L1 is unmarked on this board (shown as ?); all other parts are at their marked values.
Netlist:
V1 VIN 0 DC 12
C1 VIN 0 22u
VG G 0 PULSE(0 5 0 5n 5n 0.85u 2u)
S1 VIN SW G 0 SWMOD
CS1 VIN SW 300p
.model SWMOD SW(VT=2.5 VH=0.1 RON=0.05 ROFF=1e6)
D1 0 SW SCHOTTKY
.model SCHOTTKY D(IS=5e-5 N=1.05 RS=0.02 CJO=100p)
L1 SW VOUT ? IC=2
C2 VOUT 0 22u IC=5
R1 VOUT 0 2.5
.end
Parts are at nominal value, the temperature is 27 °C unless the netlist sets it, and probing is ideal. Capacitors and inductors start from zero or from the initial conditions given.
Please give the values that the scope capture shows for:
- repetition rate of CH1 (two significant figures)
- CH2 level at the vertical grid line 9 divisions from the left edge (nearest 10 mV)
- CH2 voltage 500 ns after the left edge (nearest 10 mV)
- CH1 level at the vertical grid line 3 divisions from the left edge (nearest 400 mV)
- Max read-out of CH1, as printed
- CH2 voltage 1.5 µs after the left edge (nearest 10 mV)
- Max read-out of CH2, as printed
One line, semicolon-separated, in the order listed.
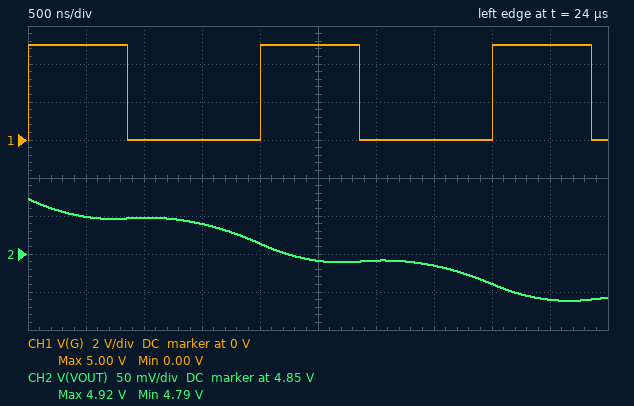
500 kHz; 4.79 V; 4.90 V; 0 V; 5.00 V; 4.89 V; 4.92 V
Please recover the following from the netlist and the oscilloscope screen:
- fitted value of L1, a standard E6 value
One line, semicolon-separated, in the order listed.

3.3 µH
